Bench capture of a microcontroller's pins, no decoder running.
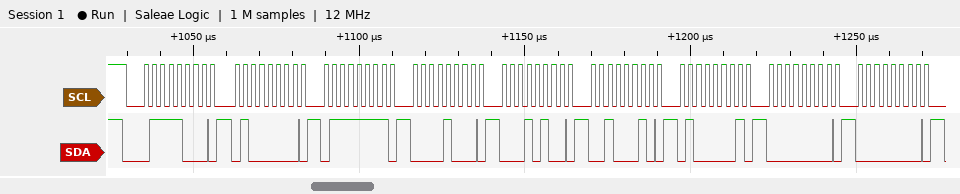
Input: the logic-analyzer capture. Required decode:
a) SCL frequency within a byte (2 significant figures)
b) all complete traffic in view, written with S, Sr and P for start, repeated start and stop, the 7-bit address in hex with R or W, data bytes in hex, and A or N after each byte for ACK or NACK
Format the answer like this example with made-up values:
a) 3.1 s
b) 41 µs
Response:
a) 400 kHz
b) S 3CW A 40 A 7F A 08 A 14 A 22 A 41 A 00 A 00 A
